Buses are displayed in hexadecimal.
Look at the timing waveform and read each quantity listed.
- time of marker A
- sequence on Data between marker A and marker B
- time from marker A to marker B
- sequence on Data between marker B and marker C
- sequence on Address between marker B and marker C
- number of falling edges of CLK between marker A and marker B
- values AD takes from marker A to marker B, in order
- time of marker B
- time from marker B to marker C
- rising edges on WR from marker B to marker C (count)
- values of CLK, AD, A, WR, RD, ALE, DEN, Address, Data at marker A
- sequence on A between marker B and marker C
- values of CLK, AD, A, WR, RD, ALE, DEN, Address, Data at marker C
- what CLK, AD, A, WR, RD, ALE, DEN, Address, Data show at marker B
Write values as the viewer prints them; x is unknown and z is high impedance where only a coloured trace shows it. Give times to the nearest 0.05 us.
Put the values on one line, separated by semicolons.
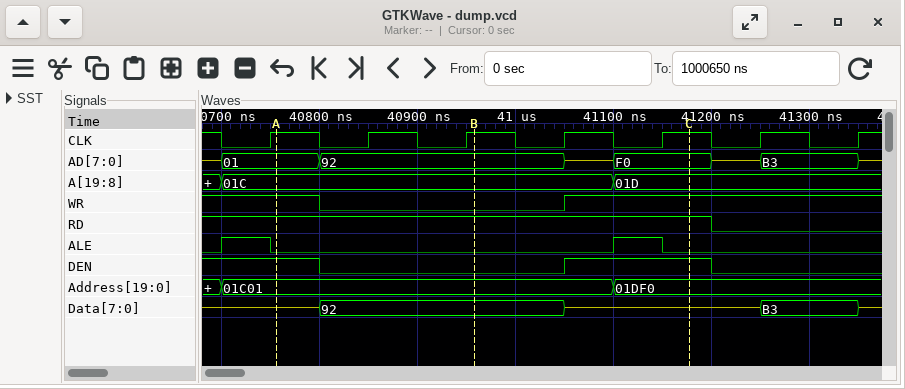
40.75 us; z, 92; 0.2 us; 92, z; 01C01, 01DF0; 2; 01, 92; 40.95 us; 0.2 us; 1; CLK=1, AD=01, A=01C, WR=1, RD=1, ALE=0, DEN=1, Address=01C01, Data=z; 01C, 01D; CLK=1, AD=F0, A=01D, WR=1, RD=1, ALE=0, DEN=1, Address=01DF0, Data=z; CLK=1, AD=92, A=01C, WR=0, RD=1, ALE=0, DEN=0, Address=01C01, Data=92
